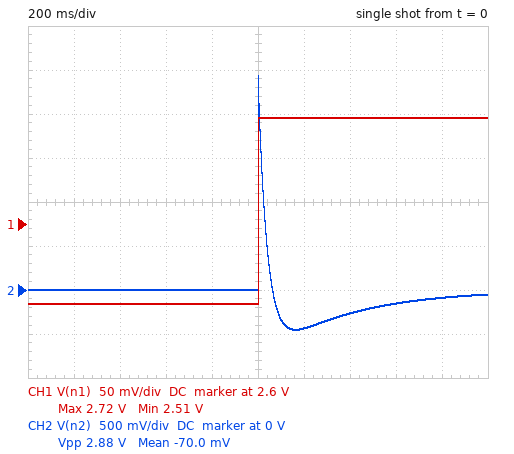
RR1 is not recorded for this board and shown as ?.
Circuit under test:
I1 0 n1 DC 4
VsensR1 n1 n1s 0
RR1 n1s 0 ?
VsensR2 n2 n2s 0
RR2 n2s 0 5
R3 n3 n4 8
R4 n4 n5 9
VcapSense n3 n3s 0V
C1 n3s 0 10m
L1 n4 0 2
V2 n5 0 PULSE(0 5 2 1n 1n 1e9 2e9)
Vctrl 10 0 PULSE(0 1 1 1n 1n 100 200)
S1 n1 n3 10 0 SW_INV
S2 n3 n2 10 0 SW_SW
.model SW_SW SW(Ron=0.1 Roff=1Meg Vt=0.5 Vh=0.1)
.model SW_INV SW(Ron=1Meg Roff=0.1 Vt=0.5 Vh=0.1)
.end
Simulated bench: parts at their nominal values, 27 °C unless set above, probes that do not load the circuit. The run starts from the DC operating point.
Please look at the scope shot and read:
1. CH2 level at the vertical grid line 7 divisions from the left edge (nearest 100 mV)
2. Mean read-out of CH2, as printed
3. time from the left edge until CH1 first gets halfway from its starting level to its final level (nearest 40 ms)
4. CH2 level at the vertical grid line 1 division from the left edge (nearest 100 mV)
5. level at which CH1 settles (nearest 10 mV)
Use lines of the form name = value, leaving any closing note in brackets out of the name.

CH2 level at the vertical grid line 7 divisions from the left edge = -300 mV
Mean read-out of CH2, as printed = -70.0 mV
time from the left edge until CH1 first gets halfway from its starting level to its final level = 1.00 s
CH2 level at the vertical grid line 1 division from the left edge = 0 V
level at which CH1 settles = 2.72 V
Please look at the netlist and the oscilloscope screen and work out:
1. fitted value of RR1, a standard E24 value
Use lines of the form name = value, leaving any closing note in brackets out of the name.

fitted value of RR1, a standard E24 value = 0.68 Ω
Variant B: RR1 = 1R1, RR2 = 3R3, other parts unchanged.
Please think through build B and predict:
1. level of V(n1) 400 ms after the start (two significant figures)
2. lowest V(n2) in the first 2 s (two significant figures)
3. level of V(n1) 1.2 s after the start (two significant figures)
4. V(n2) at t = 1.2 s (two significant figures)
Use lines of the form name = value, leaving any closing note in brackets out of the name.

level of V(n1) 400 ms after the start = 3.9 V
lowest V(n2) in the first 2 s = -530 mV
level of V(n1) 1.2 s after the start = 4.4 V
V(n2) at t = 1.2 s = -480 mV
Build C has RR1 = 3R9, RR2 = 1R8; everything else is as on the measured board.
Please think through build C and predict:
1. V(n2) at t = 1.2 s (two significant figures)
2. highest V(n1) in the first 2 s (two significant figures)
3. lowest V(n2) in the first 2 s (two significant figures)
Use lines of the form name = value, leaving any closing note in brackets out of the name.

V(n2) at t = 1.2 s = -750 mV
highest V(n1) in the first 2 s = 16 V
lowest V(n2) in the first 2 s = -920 mV
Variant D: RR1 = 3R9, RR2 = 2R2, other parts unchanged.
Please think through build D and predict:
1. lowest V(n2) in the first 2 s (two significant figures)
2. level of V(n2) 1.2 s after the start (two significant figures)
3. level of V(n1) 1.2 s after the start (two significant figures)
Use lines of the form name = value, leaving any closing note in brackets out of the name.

lowest V(n2) in the first 2 s = -1.1 V
level of V(n2) 1.2 s after the start = -910 mV
level of V(n1) 1.2 s after the start = 16 V
